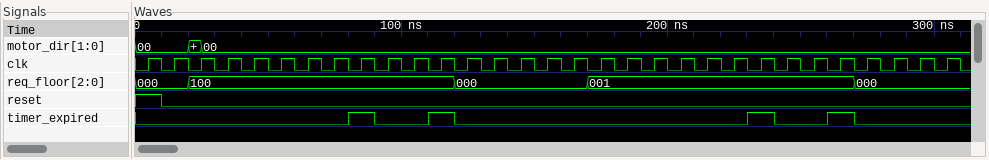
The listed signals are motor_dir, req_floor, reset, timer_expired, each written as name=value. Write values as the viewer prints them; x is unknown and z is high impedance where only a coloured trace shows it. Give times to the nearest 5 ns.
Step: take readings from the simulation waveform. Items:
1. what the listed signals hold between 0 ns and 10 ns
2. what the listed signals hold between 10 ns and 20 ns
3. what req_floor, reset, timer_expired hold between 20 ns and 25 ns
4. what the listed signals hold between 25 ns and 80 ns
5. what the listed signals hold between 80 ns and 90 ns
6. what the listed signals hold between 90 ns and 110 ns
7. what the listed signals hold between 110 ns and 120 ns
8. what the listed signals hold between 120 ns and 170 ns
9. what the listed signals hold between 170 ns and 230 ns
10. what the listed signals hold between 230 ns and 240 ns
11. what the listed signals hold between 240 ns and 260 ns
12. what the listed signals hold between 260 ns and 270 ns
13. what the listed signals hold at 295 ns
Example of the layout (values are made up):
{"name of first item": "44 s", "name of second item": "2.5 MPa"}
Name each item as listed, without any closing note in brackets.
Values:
{"what the listed signals hold between 0 ns and 10 ns": "motor_dir=00, req_floor=000, reset=1, timer_expired=0", "what the listed signals hold between 10 ns and 20 ns": "motor_dir=00, req_floor=000, reset=0, timer_expired=0", "what req_floor, reset, timer_expired hold between 20 ns and 25 ns": "req_floor=100, reset=0, timer_expired=0", "what the listed signals hold between 25 ns and 80 ns": "motor_dir=00, req_floor=100, reset=0, timer_expired=0", "what the listed signals hold between 80 ns and 90 ns": "motor_dir=00, req_floor=100, reset=0, timer_expired=1", "what the listed signals hold between 90 ns and 110 ns": "motor_dir=00, req_floor=100, reset=0, timer_expired=0", "what the listed signals hold between 110 ns and 120 ns": "motor_dir=00, req_floor=100, reset=0, timer_expired=1", "what the listed signals hold between 120 ns and 170 ns": "motor_dir=00, req_floor=000, reset=0, timer_expired=0", "what the listed signals hold between 170 ns and 230 ns": "motor_dir=00, req_floor=001, reset=0, timer_expired=0", "what the listed signals hold between 230 ns and 240 ns": "motor_dir=00, req_floor=001, reset=0, timer_expired=1", "what the listed signals hold between 240 ns and 260 ns": "motor_dir=00, req_floor=001, reset=0, timer_expired=0", "what the listed signals hold between 260 ns and 270 ns": "motor_dir=00, req_floor=001, reset=0, timer_expired=1", "what the listed signals hold at 295 ns": "motor_dir=00, req_floor=000, reset=0, timer_expired=0"}
